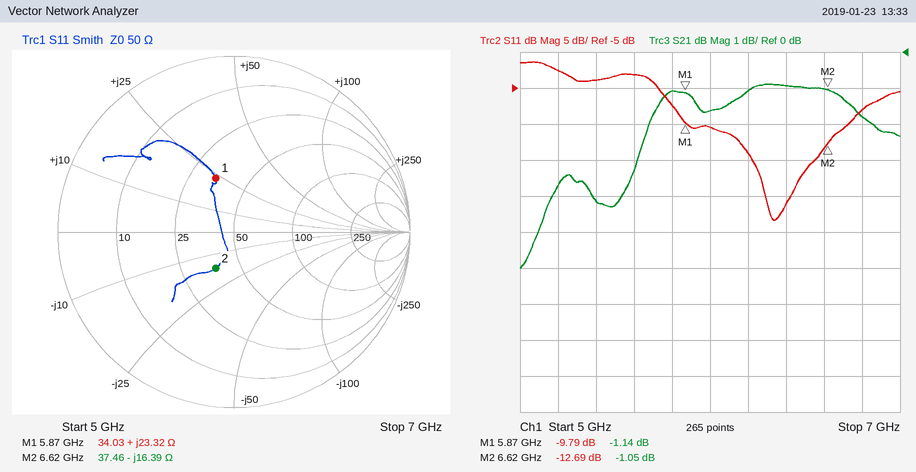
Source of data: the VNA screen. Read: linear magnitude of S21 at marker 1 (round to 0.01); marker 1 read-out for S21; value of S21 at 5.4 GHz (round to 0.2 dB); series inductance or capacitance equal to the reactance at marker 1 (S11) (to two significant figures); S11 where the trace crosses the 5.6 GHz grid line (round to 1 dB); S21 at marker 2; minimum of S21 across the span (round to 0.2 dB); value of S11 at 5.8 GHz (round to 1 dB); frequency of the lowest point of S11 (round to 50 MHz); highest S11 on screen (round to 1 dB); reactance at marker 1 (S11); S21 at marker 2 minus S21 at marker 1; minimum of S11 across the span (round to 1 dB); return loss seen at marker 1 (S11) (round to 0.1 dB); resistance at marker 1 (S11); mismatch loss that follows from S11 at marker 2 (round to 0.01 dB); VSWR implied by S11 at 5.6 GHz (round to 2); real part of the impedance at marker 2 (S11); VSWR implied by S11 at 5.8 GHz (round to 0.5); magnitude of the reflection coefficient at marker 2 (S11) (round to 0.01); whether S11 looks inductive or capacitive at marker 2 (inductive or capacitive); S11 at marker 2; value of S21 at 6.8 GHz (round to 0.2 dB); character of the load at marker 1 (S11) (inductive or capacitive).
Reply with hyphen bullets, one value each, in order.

- 0.88
- -1.14 dB
- -4.2 dB
- 630 pH
- -3 dB
- -1.05 dB
- -6.0 dB
- -7 dB
- 6.35 GHz
- -1 dB
- +23.32 Ω
- 0.09 dB
- -23 dB
- 9.8 dB
- 34.03 Ω
- 0.24 dB
- 6
- 37.46 Ω
- 2.5
- 0.23
- capacitive
- -12.69 dB
- -1.8 dB
- inductive
